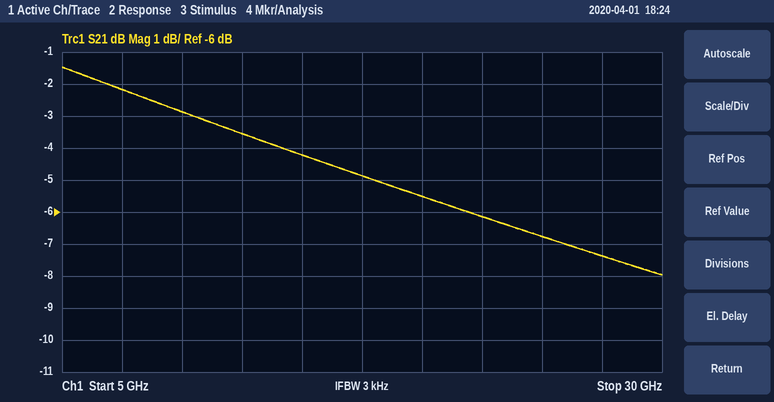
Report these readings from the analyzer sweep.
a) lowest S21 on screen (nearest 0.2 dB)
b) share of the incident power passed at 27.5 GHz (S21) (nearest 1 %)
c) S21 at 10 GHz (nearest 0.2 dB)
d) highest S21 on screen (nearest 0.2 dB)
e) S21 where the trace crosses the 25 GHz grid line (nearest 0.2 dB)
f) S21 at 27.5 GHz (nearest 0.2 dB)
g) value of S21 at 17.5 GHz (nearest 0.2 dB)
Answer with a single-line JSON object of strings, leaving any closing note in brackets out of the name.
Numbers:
{"lowest S21 on screen": "-8.0 dB", "share of the incident power passed at 27.5 GHz (S21)": "18 %", "S21 at 10 GHz": "-2.8 dB", "highest S21 on screen": "-1.4 dB", "S21 where the trace crosses the 25 GHz grid line": "-6.8 dB", "S21 at 27.5 GHz": "-7.4 dB", "value of S21 at 17.5 GHz": "-4.8 dB"}
